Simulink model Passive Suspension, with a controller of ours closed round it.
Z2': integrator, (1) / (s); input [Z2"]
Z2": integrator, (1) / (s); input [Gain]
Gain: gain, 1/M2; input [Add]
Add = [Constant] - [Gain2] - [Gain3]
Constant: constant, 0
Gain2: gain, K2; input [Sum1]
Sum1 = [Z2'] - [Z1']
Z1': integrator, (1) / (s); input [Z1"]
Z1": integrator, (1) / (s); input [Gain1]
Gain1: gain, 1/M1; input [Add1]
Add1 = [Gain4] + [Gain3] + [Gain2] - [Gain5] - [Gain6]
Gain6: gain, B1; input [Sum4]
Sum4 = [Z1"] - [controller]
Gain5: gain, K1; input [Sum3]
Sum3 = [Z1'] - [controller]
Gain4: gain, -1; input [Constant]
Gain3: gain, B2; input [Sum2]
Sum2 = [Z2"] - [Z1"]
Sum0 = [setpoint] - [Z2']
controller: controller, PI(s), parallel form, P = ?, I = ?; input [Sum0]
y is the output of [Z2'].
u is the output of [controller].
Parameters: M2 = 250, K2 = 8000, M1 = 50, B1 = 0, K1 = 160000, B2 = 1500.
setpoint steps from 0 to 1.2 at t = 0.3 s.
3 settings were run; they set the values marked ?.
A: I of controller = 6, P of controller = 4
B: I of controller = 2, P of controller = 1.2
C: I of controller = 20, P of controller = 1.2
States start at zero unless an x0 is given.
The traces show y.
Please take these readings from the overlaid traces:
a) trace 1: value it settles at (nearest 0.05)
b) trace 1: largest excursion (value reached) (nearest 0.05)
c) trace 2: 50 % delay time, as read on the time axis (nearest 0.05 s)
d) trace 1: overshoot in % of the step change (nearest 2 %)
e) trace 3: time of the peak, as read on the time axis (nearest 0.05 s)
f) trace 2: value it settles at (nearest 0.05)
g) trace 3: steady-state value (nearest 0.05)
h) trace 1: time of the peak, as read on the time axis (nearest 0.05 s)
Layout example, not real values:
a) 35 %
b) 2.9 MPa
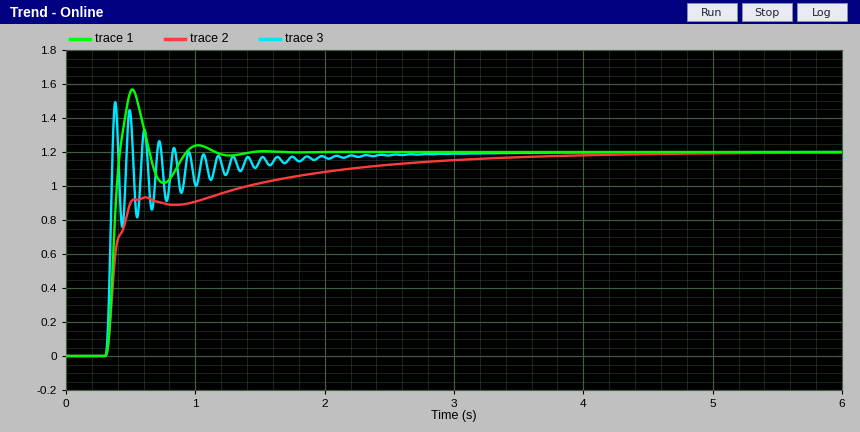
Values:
a) 1.20
b) 1.55
c) 0.40 s
d) 30 %
e) 0.40 s
f) 1.20
g) 1.20
h) 0.50 s
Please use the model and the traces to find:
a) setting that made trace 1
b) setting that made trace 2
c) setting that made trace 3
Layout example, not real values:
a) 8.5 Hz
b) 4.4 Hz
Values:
a) C
b) B
c) A
